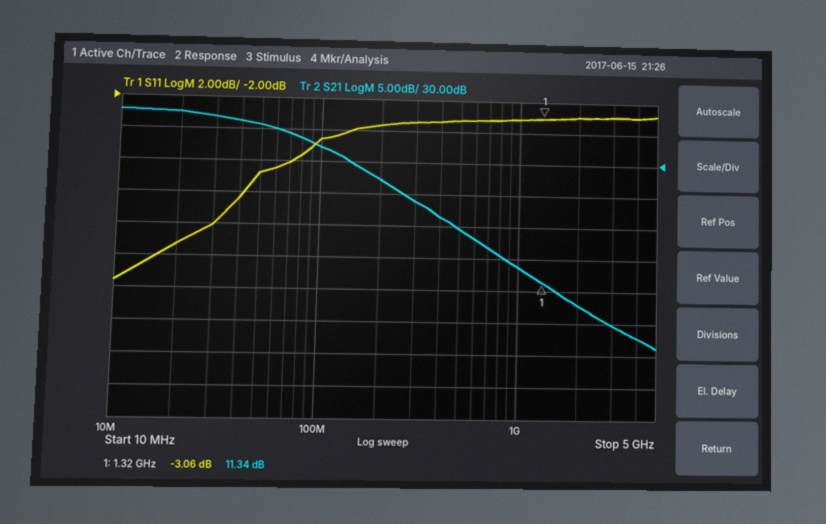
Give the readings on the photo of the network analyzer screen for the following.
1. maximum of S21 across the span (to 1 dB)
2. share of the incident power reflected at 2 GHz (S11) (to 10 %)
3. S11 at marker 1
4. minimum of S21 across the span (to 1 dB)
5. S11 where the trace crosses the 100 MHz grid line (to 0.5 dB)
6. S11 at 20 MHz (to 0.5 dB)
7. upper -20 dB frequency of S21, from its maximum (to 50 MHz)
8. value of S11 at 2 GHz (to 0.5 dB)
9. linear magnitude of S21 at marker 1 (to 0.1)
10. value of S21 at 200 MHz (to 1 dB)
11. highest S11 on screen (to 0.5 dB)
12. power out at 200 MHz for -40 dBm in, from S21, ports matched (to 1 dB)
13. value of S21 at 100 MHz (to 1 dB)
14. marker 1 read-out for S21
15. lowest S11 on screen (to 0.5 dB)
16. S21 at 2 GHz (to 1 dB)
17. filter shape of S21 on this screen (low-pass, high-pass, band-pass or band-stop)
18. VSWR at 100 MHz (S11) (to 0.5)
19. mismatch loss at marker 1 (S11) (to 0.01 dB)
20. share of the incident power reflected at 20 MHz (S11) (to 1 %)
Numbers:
38 dB
50 %
-3.06 dB
1 dB
-4.5 dB
-11.5 dB
600 MHz
-3.0 dB
3.7
27 dB
-3.0 dB
-13 dBm
32 dB
11.34 dB
-13.5 dB
8 dB
low-pass
4.0
2.96 dB
7 %
